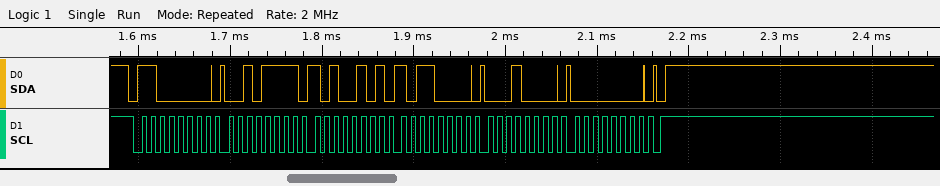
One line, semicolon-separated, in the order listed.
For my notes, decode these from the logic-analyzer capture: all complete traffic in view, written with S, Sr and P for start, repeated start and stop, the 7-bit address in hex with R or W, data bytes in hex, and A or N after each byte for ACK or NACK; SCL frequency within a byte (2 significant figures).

S 60W A 2F A A5 A B0 A 10 A 00 A P; 100 kHz
